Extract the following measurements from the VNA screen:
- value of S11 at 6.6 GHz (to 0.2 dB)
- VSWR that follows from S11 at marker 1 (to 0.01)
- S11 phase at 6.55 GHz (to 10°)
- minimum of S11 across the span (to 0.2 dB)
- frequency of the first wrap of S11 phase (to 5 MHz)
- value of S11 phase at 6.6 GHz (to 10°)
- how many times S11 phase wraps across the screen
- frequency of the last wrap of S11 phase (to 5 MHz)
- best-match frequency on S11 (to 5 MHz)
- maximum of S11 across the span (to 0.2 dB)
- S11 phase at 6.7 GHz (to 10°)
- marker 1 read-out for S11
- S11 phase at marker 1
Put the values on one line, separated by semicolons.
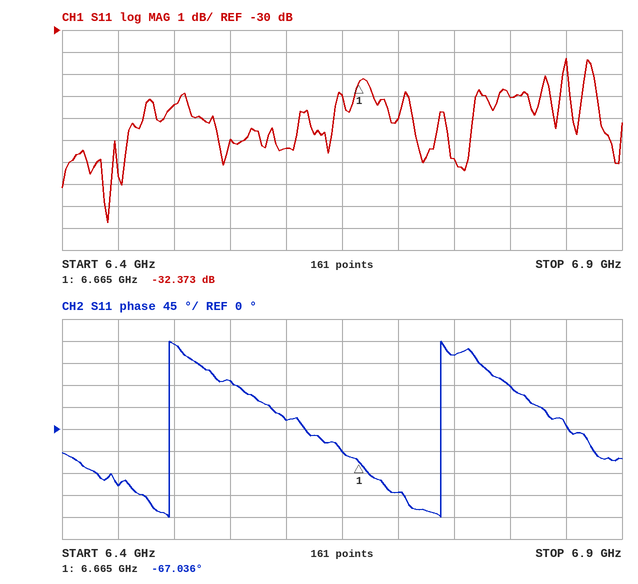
-35.4 dB; 1.05; 100°; -38.8 dB; 6.495 GHz; 20°; 2; 6.740 GHz; 6.440 GHz; -31.2 dB; -130°; -32.373 dB; -67.036°
